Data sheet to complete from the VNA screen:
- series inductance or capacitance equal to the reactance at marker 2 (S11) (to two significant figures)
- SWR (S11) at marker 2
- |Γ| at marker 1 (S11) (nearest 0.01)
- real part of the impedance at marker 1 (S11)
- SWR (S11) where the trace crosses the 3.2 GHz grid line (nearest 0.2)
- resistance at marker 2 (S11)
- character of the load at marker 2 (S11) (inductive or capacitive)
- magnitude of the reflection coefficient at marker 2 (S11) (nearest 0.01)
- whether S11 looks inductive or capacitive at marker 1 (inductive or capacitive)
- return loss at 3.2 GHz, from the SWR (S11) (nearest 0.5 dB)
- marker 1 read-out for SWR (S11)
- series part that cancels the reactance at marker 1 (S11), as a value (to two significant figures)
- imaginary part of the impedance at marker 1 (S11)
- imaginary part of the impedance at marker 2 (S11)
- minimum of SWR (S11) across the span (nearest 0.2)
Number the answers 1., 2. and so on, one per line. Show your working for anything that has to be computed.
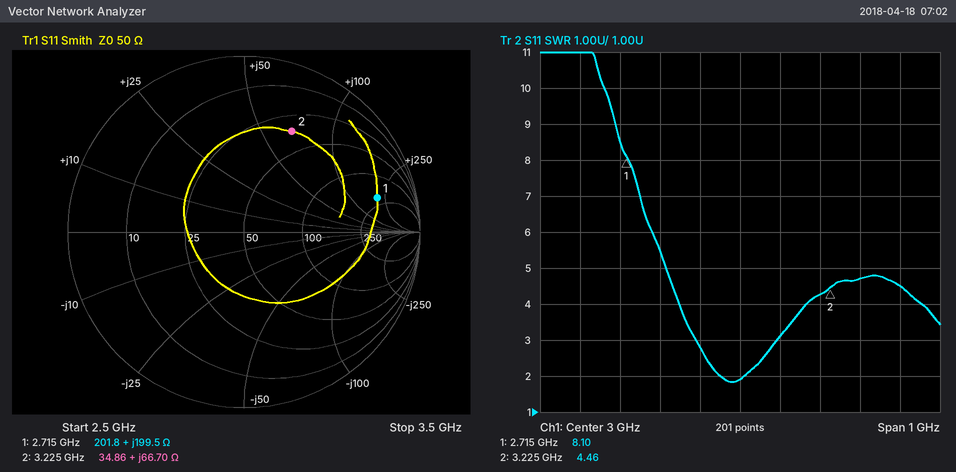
1. L = 66.7 Ω/(2π × 3.225 GHz) ≈ 3.3 nH
2. 4.46
3. 0.78
4. 201.8 Ω
5. 4.2
6. 34.86 Ω
7. inductive
8. 0.63
9. inductive
10. −20 log10((4.2 − 1)/(4.2 + 1)) ≈ 4.22 dB, so 4.0 dB to the nearest 0.5 dB
11. 8.10
12. C = 1/(2π × 2.715 GHz × 199.5 Ω) ≈ 294 fF, so 290 fF to two significant figures
13. +199.5 Ω
14. +66.70 Ω
15. 1.8
